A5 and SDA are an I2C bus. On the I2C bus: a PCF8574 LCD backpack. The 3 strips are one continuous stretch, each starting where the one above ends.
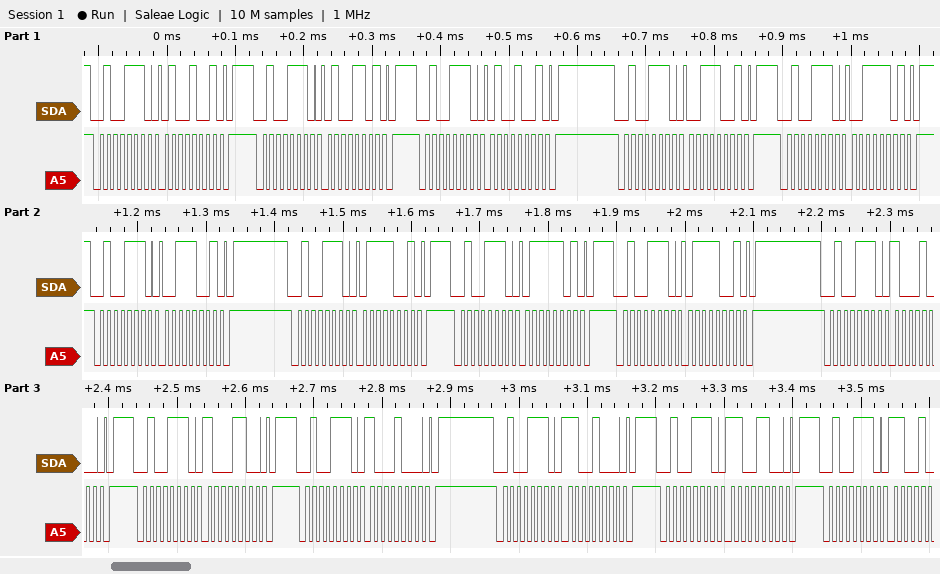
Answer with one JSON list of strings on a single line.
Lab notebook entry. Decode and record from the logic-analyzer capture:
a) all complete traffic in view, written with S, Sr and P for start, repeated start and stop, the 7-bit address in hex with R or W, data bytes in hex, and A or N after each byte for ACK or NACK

["S 27W A 49 A P S 27W A 4D A P S 27W A 49 A P S 27W A 39 A P S 27W A 3D A P S 27W A 39 A P S 27W A 79 A P S 27W A 7D A P S 27W A 79 A P S 27W A 88 A P S 27W A 8C A P S 27W A 88 A P S 27W A C8 A P S 27W A CC A P S 27W A"]
